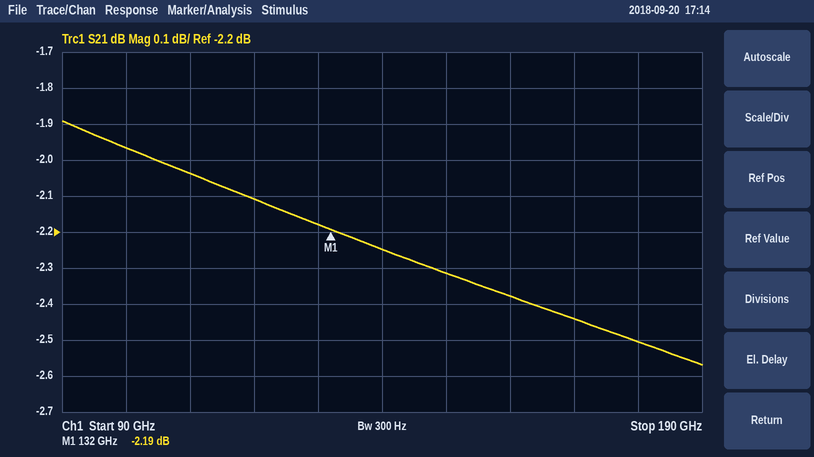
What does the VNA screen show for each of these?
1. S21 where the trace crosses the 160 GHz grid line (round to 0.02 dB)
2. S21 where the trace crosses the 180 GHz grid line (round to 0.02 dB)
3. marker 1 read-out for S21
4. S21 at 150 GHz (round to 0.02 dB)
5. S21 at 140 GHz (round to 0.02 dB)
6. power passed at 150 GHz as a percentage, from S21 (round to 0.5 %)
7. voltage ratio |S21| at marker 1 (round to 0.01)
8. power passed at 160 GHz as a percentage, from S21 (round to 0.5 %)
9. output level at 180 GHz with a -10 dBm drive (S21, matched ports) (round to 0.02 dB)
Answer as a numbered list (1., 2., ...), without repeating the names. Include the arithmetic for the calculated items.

1. -2.38 dB
2. -2.50 dB
3. -2.19 dB
4. -2.32 dB
5. -2.24 dB
6. 10^(-2.32/10) ≈ 58.6 %, so 58.5 % to the nearest 0.5 %
7. 10^(-2.19/20) ≈ 0.78
8. 10^(-2.38/10) ≈ 57.8 %, so 58.0 % to the nearest 0.5 %
9. -10 dBm + (-2.50 dB) = -12.50 dBm
